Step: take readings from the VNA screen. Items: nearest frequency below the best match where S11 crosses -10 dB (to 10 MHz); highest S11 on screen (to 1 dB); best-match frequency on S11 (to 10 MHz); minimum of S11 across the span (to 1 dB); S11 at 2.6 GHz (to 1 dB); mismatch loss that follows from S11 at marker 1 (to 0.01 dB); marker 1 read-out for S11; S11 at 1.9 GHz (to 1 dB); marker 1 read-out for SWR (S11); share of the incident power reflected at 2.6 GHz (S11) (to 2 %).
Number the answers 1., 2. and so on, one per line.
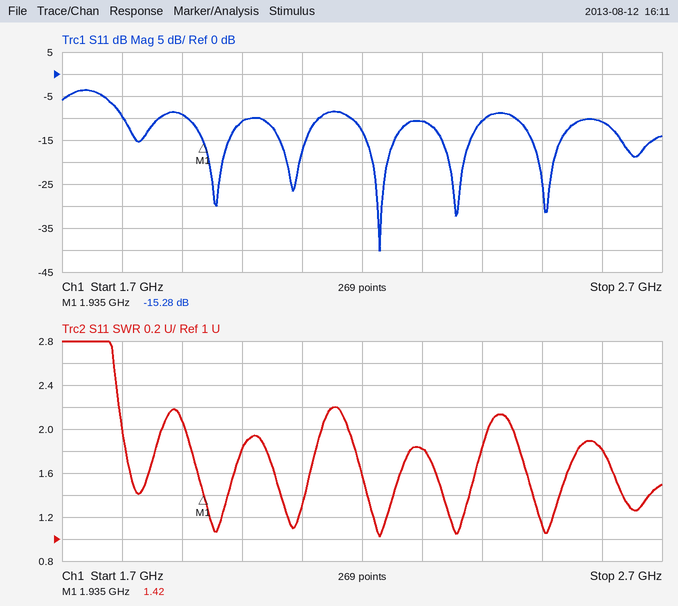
1. 2.18 GHz
2. -4 dB
3. 2.23 GHz
4. -40 dB
5. -11 dB
6. 0.13 dB
7. -15.28 dB
8. -9 dB
9. 1.42
10. 8 %
